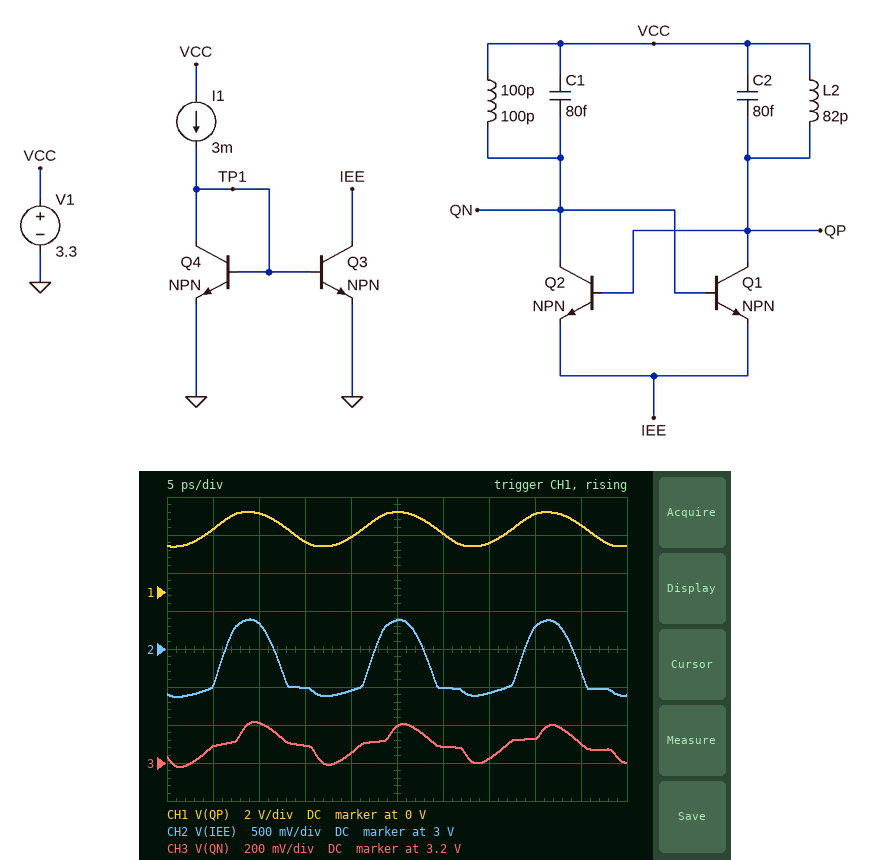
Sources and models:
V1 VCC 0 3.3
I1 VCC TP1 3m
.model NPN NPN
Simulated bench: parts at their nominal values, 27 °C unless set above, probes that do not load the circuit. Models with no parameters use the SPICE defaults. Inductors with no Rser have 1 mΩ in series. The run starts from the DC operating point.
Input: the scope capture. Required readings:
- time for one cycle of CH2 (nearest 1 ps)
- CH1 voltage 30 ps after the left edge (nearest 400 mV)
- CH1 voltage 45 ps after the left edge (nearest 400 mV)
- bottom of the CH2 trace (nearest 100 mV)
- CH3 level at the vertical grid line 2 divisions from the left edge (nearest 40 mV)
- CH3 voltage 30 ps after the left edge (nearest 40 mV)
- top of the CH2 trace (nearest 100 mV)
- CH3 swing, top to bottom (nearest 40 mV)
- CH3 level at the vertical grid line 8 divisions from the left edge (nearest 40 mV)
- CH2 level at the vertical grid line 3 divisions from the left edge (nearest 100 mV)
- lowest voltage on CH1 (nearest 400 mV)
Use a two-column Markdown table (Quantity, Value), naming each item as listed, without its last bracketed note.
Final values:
| Quantity | Value |
|---|---|
| time for one cycle of CH2 | 16 ps |
| CH1 voltage 30 ps after the left edge | 3.2 V |
| CH1 voltage 45 ps after the left edge | 3.6 V |
| bottom of the CH2 trace | 2.4 V |
| CH3 level at the vertical grid line 2 divisions from the left edge | 3.40 V |
| CH3 voltage 30 ps after the left edge | 3.28 V |
| top of the CH2 trace | 3.4 V |
| CH3 swing, top to bottom | 240 mV |
| CH3 level at the vertical grid line 8 divisions from the left edge | 3.32 V |
| CH2 level at the vertical grid line 3 divisions from the left edge | 2.5 V |
| lowest voltage on CH1 | 2.4 V |
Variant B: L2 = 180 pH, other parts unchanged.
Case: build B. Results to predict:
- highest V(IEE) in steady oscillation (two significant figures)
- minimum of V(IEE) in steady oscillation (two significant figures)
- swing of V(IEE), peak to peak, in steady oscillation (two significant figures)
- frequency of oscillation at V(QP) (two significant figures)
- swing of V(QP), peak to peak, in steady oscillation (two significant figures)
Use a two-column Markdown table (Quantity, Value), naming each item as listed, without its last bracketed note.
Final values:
| Quantity | Value |
|---|---|
| highest V(IEE) in steady oscillation | 3.4 V |
| minimum of V(IEE) in steady oscillation | 2.3 V |
| swing of V(IEE), peak to peak, in steady oscillation | 1.2 V |
| frequency of oscillation at V(QP) | 41 GHz |
| swing of V(QP), peak to peak, in steady oscillation | 1.9 V |
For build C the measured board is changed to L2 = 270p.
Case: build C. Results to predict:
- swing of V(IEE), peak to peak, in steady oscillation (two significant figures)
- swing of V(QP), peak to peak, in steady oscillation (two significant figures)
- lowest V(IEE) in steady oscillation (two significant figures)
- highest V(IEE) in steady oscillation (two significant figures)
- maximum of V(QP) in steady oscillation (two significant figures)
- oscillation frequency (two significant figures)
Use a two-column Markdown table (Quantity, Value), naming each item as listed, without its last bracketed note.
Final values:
| Quantity | Value |
|---|---|
| swing of V(IEE), peak to peak, in steady oscillation | 820 mV |
| swing of V(QP), peak to peak, in steady oscillation | 1.6 V |
| lowest V(IEE) in steady oscillation | 2.5 V |
| highest V(IEE) in steady oscillation | 3.3 V |
| maximum of V(QP) in steady oscillation | 4.1 V |
| oscillation frequency | 33 GHz |
